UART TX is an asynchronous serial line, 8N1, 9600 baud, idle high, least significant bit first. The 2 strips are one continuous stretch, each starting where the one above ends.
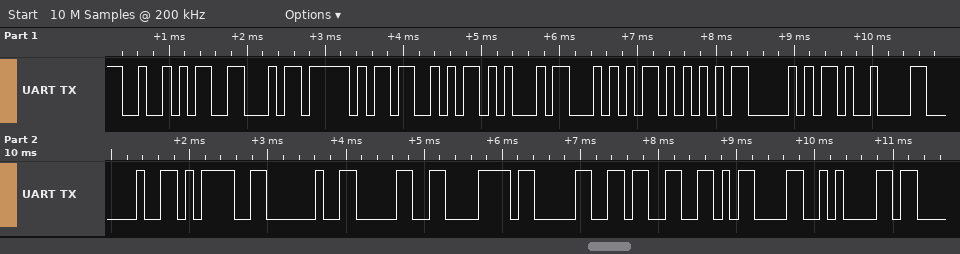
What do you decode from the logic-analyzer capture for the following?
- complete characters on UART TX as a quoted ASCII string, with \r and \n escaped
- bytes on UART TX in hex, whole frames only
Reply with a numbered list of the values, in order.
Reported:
1. "RF_SETUP\t = 0x03\r\n"
2. 52 46 5F 53 45 54 55 50 09 20 3D 20 30 78 30 33 0D 0A
